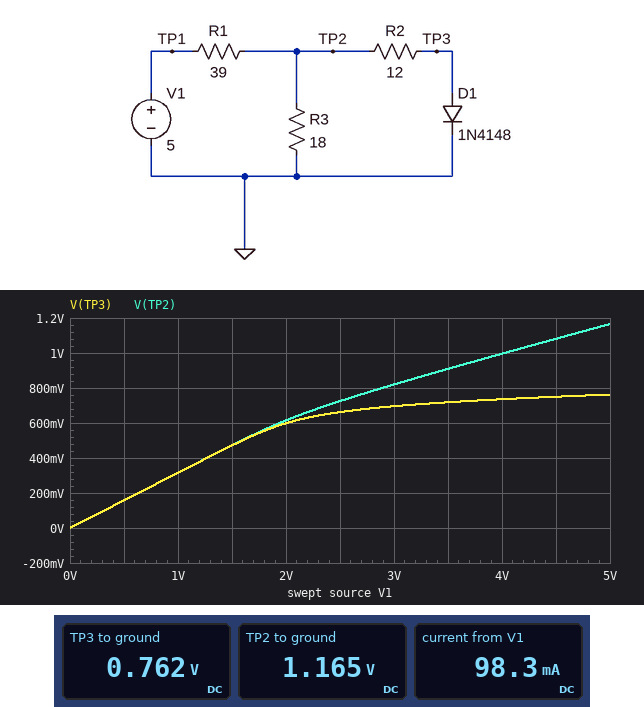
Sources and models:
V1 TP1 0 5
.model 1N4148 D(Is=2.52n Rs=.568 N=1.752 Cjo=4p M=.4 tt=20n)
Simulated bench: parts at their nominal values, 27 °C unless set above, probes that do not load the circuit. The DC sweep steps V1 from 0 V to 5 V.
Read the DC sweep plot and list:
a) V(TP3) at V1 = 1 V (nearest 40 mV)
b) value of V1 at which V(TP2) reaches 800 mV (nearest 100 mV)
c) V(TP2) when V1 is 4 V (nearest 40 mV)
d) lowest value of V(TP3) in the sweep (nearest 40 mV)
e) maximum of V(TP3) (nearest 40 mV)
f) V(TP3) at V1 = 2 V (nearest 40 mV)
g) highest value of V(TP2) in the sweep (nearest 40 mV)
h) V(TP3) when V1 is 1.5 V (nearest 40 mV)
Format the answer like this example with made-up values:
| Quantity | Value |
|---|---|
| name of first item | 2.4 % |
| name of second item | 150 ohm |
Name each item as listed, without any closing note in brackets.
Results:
| Quantity | Value |
|---|---|
| V(TP3) at V1 = 1 V | 320 mV |
| value of V1 at which V(TP2) reaches 800 mV | 2.9 V |
| V(TP2) when V1 is 4 V | 1.00 V |
| lowest value of V(TP3) in the sweep | 0 V |
| maximum of V(TP3) | 760 mV |
| V(TP3) at V1 = 2 V | 600 mV |
| highest value of V(TP2) in the sweep | 1.16 V |
| V(TP3) when V1 is 1.5 V | 480 mV |
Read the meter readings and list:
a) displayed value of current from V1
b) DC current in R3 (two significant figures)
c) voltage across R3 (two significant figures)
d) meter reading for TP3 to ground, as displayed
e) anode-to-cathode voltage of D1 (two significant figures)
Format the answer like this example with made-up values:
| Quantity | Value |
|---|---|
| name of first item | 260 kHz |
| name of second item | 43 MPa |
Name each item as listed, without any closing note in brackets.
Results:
| Quantity | Value |
|---|---|
| displayed value of current from V1 | 98.3 mA |
| DC current in R3 | 65 mA |
| voltage across R3 | 1.2 V |
| meter reading for TP3 to ground, as displayed | 0.762 V |
| anode-to-cathode voltage of D1 | 760 mV |
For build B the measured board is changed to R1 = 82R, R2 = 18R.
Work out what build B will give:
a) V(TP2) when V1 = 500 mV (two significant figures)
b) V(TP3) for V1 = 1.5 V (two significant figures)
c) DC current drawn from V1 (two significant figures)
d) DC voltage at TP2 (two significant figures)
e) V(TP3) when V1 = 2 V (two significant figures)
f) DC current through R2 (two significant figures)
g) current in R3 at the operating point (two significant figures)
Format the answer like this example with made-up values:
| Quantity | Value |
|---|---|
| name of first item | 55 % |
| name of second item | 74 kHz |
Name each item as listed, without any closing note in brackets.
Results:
| Quantity | Value |
|---|---|
| V(TP2) when V1 = 500 mV | 90 mV |
| V(TP3) for V1 = 1.5 V | 270 mV |
| DC current drawn from V1 | 51 mA |
| DC voltage at TP2 | 800 mV |
| V(TP3) when V1 = 2 V | 360 mV |
| DC current through R2 | 6.9 mA |
| current in R3 at the operating point | 44 mA |
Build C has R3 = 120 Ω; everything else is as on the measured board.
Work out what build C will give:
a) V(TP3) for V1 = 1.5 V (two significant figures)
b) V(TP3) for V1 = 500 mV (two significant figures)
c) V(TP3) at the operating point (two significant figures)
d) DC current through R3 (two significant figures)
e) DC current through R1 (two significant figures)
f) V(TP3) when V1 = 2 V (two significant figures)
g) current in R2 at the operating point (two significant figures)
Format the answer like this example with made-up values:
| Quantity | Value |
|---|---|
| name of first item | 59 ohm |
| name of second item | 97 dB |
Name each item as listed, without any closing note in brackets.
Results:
| Quantity | Value |
|---|---|
| V(TP3) for V1 = 1.5 V | 700 mV |
| V(TP3) for V1 = 500 mV | 380 mV |
| V(TP3) at the operating point | 820 mV |
| DC current through R3 | 14 mA |
| DC current through R1 | 85 mA |
| V(TP3) when V1 = 2 V | 730 mV |
| current in R2 at the operating point | 71 mA |
